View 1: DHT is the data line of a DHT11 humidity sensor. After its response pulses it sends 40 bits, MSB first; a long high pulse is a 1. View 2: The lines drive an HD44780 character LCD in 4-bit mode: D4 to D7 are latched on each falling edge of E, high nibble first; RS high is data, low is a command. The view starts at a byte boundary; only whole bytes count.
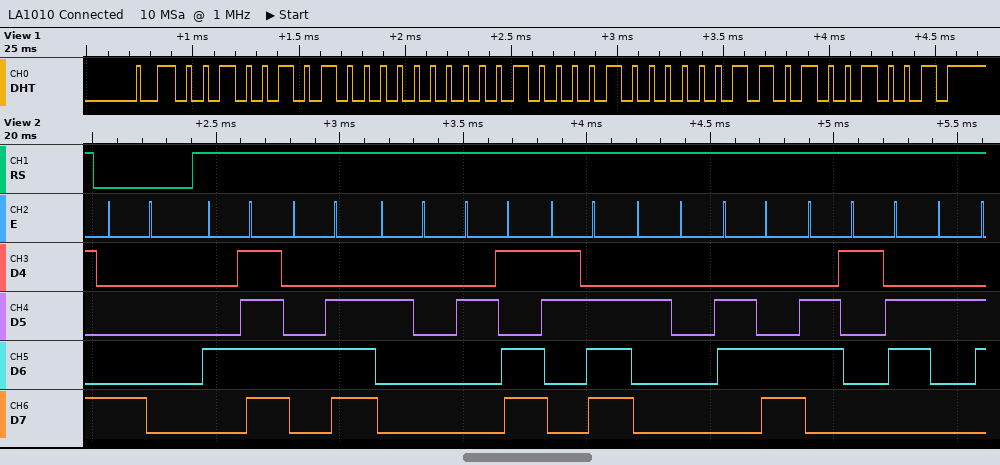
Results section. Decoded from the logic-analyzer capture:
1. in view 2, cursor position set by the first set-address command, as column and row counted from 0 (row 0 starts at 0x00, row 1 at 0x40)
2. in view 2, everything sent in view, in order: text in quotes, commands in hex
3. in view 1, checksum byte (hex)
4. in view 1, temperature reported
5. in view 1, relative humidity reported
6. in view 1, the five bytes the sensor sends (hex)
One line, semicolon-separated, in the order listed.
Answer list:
column 0, row 0; 0x80 "ON -> lab"; 0x49; 33.3 °C; 37 %; 25 00 21 03 49
